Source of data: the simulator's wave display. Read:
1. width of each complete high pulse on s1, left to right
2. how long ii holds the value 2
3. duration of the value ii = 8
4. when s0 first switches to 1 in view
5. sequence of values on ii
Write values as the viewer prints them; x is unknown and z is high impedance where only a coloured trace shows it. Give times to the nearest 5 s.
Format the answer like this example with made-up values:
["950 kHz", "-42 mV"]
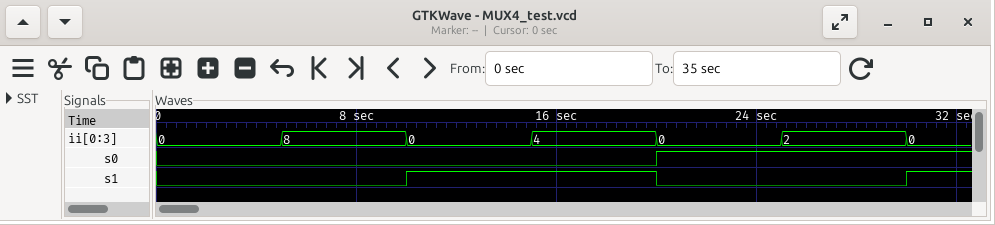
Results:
["10 s", "5 s", "5 s", "20 s", "0, 8, 0, 4, 0, 2, 0"]
